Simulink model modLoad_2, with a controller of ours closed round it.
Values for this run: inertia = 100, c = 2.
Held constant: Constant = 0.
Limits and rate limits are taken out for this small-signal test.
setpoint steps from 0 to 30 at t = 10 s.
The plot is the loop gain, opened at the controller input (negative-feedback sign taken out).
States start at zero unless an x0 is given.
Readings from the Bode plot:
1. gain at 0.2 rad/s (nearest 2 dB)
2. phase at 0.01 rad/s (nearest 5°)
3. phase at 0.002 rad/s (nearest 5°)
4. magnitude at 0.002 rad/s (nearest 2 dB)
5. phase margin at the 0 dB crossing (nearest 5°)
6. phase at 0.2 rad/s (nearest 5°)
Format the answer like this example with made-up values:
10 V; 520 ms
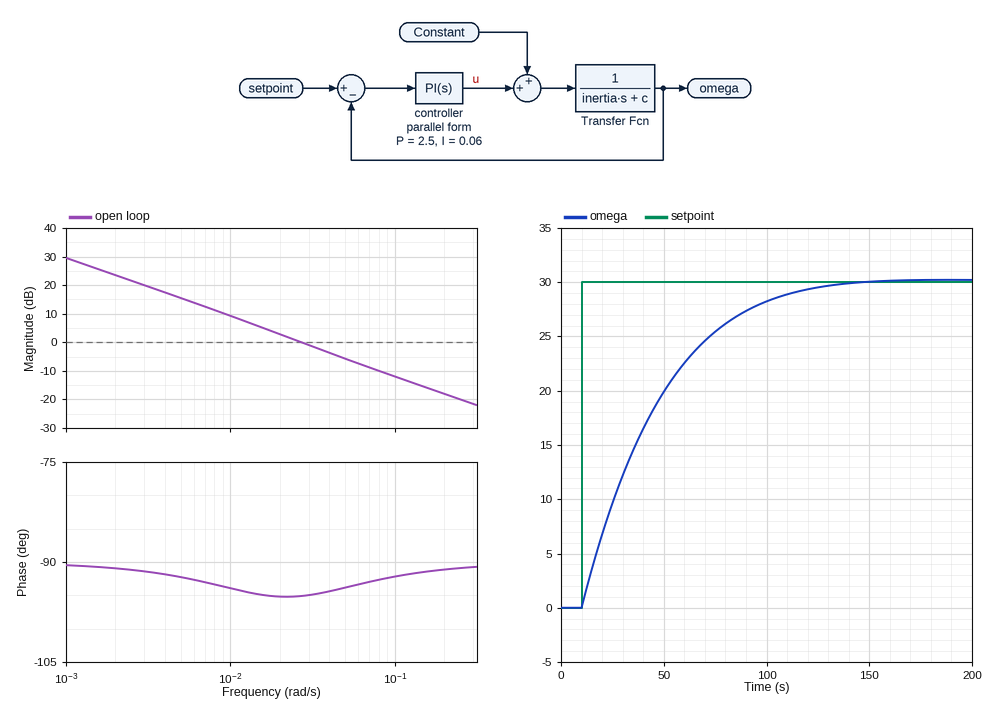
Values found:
-18 dB; -95°; -90°; 24 dB; 85°; -90°
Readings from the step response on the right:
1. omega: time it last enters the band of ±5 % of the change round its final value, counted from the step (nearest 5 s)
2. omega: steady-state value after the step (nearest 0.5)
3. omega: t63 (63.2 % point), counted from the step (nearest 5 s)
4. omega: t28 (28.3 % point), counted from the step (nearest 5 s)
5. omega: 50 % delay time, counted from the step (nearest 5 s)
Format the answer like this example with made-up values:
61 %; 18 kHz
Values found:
95 s; 30.0; 35 s; 15 s; 25 s
